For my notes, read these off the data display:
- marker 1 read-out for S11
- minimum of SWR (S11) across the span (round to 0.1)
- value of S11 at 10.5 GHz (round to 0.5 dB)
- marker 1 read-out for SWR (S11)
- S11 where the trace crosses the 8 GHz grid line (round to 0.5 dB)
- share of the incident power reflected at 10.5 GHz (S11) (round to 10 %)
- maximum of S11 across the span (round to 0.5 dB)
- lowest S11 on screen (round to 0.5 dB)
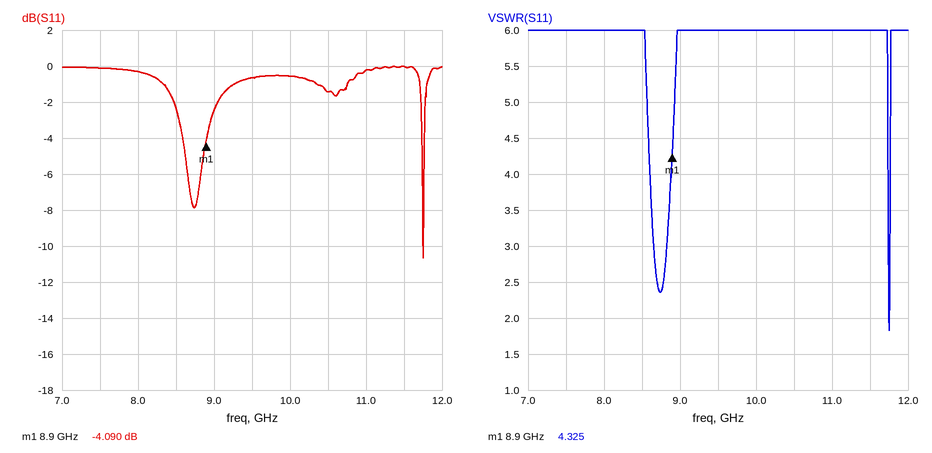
-4.090 dB
1.8
-1.5 dB
4.325
-0.5 dB
70 %
0.0 dB
-10.5 dB
